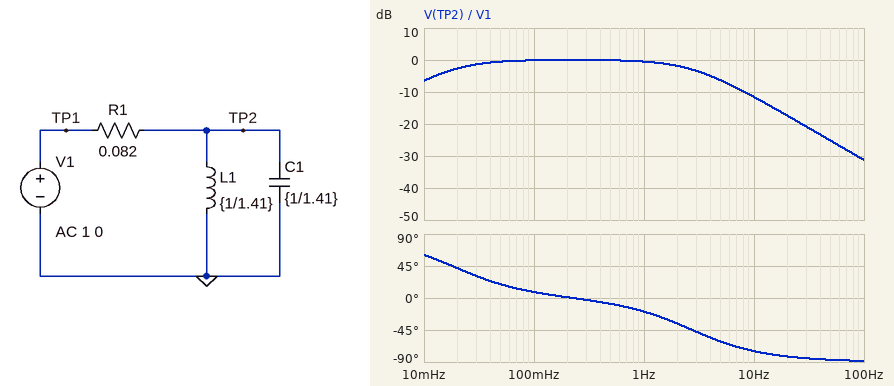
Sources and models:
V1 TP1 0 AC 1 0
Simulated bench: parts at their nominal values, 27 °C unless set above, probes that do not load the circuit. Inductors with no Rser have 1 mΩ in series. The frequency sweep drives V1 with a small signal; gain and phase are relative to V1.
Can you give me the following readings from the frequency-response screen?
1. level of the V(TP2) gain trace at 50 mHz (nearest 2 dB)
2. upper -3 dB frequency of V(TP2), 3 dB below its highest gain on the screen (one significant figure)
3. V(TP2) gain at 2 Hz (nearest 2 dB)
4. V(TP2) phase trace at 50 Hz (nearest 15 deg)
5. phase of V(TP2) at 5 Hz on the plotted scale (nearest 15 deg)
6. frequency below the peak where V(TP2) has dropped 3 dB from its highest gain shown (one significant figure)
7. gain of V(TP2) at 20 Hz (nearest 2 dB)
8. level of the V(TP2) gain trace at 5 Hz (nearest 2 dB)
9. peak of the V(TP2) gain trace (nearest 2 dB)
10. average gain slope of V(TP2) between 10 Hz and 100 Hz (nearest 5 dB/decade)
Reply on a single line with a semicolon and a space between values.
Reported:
0 dB; 3 Hz; -2 dB; -90 deg; -60 deg; 20 mHz; -18 dB; -6 dB; 0 dB; -20 dB/decade
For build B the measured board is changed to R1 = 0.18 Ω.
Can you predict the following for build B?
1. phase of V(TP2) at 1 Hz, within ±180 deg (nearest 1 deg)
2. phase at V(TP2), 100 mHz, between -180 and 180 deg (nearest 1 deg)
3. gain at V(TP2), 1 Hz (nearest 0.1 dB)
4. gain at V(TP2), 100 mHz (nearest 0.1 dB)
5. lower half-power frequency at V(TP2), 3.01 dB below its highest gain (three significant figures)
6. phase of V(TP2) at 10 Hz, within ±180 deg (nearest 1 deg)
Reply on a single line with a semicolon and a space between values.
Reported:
-37 deg; 18 deg; -2.0 dB; -0.4 dB; 39.4 mHz; -83 deg
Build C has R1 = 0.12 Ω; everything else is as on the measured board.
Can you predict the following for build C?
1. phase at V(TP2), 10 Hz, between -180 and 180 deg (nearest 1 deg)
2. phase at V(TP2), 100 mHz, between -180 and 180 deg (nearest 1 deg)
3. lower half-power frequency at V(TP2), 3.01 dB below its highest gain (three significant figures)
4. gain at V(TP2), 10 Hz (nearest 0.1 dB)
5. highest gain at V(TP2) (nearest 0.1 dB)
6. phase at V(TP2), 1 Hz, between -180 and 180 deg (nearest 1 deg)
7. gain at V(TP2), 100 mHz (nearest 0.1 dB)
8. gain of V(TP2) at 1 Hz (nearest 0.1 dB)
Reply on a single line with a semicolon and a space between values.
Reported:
-79 deg; 12 deg; 26.8 mHz; -14.7 dB; 0 dB; -27 deg; -0.2 dB; -1.0 dB
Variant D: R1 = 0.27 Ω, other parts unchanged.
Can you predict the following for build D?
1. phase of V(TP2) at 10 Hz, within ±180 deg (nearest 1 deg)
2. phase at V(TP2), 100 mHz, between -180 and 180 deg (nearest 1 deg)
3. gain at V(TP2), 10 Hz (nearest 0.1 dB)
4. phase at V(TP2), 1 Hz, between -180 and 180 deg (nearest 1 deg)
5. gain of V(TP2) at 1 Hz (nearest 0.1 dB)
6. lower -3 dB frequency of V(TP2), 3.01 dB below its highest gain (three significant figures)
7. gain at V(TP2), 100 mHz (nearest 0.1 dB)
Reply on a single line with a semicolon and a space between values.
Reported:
-85 deg; 26 deg; -21.6 dB; -49 deg; -3.6 dB; 56.9 mHz; -0.9 dB
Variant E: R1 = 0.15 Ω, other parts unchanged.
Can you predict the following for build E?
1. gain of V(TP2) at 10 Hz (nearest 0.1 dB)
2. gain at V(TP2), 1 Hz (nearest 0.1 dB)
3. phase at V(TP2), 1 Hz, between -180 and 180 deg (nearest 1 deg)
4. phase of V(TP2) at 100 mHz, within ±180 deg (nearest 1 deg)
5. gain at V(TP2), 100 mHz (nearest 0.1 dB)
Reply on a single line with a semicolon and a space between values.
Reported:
-16.6 dB; -1.5 dB; -32 deg; 15 deg; -0.3 dB
